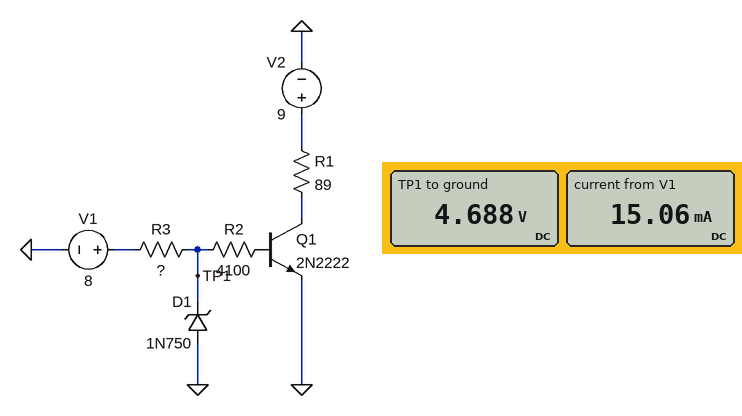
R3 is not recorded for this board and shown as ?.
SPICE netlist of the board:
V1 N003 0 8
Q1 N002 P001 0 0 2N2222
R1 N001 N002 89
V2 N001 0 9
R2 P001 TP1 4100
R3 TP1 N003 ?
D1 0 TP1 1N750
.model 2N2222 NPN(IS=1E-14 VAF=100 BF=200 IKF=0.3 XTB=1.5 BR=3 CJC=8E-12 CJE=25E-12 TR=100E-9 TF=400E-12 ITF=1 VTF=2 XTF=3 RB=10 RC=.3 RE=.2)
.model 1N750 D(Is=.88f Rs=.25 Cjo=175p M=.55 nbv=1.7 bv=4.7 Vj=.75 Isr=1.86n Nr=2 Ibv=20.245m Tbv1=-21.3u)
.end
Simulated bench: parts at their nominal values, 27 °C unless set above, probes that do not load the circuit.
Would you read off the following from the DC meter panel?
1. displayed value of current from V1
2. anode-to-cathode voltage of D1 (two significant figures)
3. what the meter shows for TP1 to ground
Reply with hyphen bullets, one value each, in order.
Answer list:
- 15.06 mA
- -4.7 V
- 4.688 V
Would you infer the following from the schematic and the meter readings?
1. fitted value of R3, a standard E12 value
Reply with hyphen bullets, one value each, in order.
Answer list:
- 220 Ω
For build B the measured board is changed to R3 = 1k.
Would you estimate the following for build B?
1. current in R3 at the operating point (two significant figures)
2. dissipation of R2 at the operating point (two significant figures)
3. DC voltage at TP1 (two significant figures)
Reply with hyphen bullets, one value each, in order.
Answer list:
- 3.4 mA
- 3.5 mW
- 4.6 V
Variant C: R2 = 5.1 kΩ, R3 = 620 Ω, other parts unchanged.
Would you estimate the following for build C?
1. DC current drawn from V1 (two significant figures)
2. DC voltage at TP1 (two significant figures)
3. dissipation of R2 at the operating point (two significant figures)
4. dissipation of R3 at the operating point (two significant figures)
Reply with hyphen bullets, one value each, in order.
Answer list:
- 5.4 mA
- 4.6 V
- 2.9 mW
- 18 mW
